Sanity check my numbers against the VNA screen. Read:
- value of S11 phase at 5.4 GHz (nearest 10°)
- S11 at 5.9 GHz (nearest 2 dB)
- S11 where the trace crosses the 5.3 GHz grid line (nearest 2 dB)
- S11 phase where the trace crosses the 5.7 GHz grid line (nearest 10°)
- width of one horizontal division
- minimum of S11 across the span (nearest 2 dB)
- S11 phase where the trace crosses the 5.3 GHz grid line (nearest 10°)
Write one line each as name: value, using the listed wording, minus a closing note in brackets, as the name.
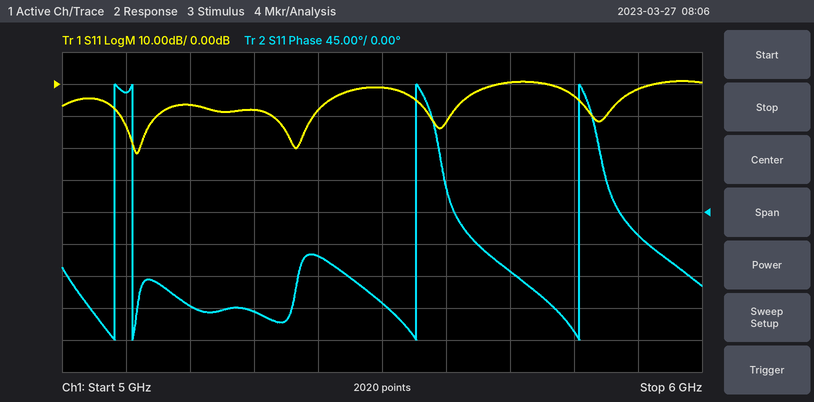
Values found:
value of S11 phase at 5.4 GHz: -60°
S11 at 5.9 GHz: -2 dB
S11 where the trace crosses the 5.3 GHz grid line: -8 dB
S11 phase where the trace crosses the 5.7 GHz grid line: -80°
width of one horizontal division: 100 MHz
minimum of S11 across the span: -22 dB
S11 phase where the trace crosses the 5.3 GHz grid line: -140°
